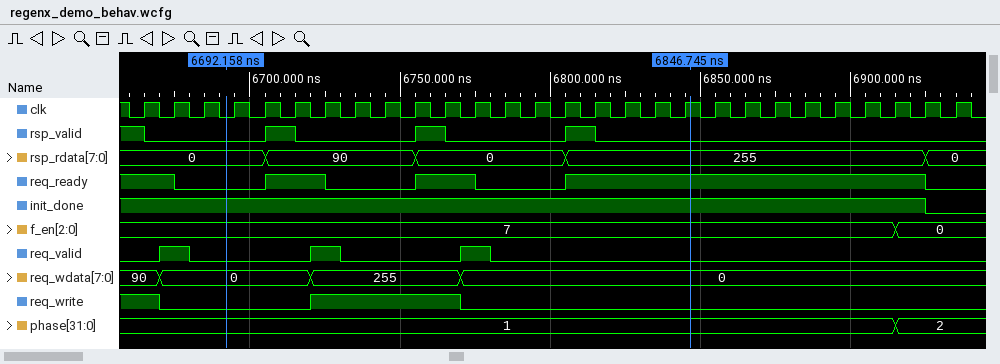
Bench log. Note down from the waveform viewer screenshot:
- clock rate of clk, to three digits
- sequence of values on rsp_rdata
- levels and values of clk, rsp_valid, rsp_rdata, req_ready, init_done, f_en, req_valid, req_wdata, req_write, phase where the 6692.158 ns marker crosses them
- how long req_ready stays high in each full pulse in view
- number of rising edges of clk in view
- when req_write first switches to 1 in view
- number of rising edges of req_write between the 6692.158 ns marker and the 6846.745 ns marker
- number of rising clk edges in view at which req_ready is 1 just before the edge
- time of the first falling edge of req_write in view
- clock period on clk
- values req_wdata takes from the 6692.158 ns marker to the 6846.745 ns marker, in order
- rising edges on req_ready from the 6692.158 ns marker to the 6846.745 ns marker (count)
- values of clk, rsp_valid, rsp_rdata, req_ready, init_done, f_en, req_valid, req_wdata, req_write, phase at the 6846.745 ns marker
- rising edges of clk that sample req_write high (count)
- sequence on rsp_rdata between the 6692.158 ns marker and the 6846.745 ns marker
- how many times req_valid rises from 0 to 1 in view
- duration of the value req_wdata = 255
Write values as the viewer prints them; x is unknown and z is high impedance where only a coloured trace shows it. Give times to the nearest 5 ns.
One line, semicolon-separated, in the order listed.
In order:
100 MHz; 0, 90, 0, 255, 0; clk=0, rsp_valid=0, rsp_rdata=0, req_ready=0, init_done=1, f_en=7, req_valid=0, req_wdata=0, req_write=0, phase=1; 20 ns, 20 ns, 120 ns; 28; 6720 ns; 1; 18; 6670 ns; 10 ns; 0, 255, 0; 3; clk=1, rsp_valid=0, rsp_rdata=255, req_ready=1, init_done=1, f_en=7, req_valid=0, req_wdata=0, req_write=0, phase=1; 6; 0, 90, 0, 255; 3; 50 ns
